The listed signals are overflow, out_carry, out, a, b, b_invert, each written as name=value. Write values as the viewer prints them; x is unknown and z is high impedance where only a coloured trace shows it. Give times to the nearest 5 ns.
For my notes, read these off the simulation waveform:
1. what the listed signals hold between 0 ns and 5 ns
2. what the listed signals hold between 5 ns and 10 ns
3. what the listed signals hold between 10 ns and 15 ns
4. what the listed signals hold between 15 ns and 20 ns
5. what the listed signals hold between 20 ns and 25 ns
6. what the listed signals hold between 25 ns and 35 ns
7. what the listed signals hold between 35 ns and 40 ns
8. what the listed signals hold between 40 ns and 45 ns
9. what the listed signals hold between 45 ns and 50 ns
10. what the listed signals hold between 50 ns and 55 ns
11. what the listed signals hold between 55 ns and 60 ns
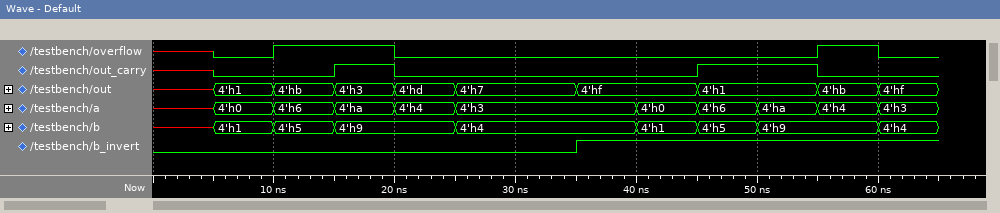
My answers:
overflow=x, out_carry=x, out=x, a=x, b=x, b_invert=0
overflow=0, out_carry=0, out=4'h1, a=4'h0, b=4'h1, b_invert=0
overflow=1, out_carry=0, out=4'hb, a=4'h6, b=4'h5, b_invert=0
overflow=1, out_carry=1, out=4'h3, a=4'ha, b=4'h9, b_invert=0
overflow=0, out_carry=0, out=4'hd, a=4'h4, b=4'h9, b_invert=0
overflow=0, out_carry=0, out=4'h7, a=4'h3, b=4'h4, b_invert=0
overflow=0, out_carry=0, out=4'hf, a=4'h3, b=4'h4, b_invert=1
overflow=0, out_carry=0, out=4'hf, a=4'h0, b=4'h1, b_invert=1
overflow=0, out_carry=1, out=4'h1, a=4'h6, b=4'h5, b_invert=1
overflow=0, out_carry=1, out=4'h1, a=4'ha, b=4'h9, b_invert=1
overflow=1, out_carry=0, out=4'hb, a=4'h4, b=4'h9, b_invert=1
